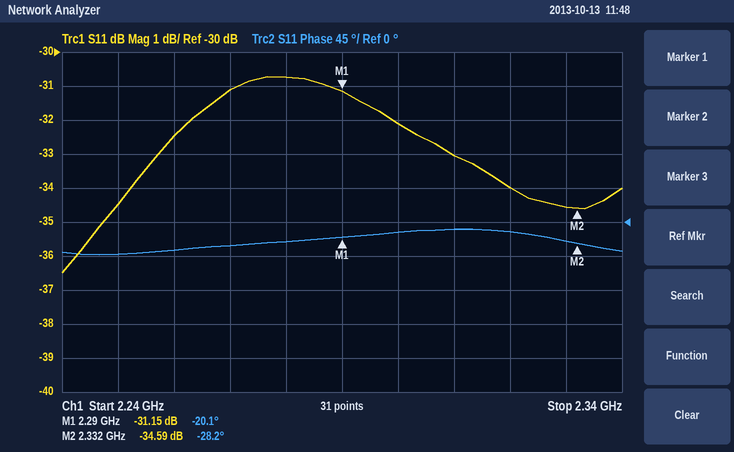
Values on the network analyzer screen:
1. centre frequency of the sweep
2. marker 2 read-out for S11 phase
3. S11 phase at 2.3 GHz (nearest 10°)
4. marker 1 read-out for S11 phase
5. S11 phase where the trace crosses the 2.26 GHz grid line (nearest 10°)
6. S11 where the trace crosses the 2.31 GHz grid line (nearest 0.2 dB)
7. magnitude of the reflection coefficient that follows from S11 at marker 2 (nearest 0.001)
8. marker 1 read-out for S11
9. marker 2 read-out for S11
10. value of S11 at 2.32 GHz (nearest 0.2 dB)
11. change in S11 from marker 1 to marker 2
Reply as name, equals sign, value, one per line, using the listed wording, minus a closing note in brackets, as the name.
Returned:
centre frequency of the sweep = 2.29 GHz
marker 2 read-out for S11 phase = -28.2°
S11 phase at 2.3 GHz = -10°
marker 1 read-out for S11 phase = -20.1°
S11 phase where the trace crosses the 2.26 GHz grid line = -40°
S11 where the trace crosses the 2.31 GHz grid line = -33.0 dB
magnitude of the reflection coefficient that follows from S11 at marker 2 = 0.019
marker 1 read-out for S11 = -31.15 dB
marker 2 read-out for S11 = -34.59 dB
value of S11 at 2.32 GHz = -34.0 dB
change in S11 from marker 1 to marker 2 = -3.44 dB
